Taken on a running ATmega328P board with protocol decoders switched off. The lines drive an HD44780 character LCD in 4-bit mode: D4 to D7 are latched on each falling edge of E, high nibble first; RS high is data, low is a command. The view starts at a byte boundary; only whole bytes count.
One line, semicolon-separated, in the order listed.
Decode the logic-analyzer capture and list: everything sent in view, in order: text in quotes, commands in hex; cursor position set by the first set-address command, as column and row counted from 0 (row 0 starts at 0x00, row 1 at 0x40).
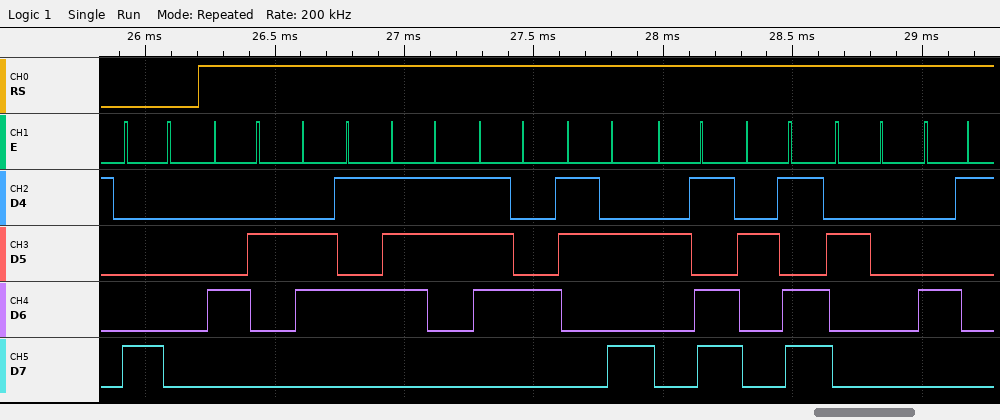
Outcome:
0x80 "Best:-- A"; column 0, row 0
